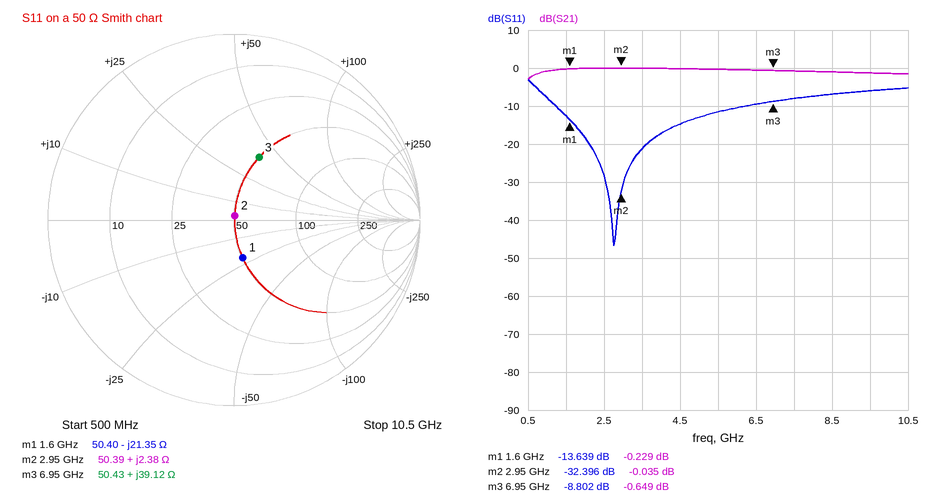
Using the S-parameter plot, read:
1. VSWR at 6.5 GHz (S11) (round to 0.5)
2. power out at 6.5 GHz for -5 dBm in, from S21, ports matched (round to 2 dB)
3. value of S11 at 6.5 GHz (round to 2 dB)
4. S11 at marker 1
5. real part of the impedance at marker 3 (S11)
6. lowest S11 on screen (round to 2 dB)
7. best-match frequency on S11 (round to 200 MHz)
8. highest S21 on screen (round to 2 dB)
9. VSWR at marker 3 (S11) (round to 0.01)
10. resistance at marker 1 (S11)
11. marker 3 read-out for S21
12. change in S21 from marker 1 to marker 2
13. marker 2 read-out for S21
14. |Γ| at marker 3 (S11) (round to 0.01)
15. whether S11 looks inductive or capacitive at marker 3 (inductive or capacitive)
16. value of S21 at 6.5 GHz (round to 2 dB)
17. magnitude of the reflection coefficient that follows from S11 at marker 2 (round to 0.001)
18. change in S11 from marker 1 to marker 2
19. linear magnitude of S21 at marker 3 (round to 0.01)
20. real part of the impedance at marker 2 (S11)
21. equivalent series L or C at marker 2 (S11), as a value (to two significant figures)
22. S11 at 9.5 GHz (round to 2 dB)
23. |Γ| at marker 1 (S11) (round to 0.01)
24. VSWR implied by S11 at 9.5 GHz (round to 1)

2.0
-6 dBm
-10 dB
-13.639 dB
50.43 Ω
-46 dB
2.8 GHz
0 dB
2.14
50.40 Ω
-0.649 dB
0.194 dB
-0.035 dB
0.36
inductive
0 dB
0.024
-18.757 dB
0.93
50.39 Ω
130 pH
-6 dB
0.21
3
